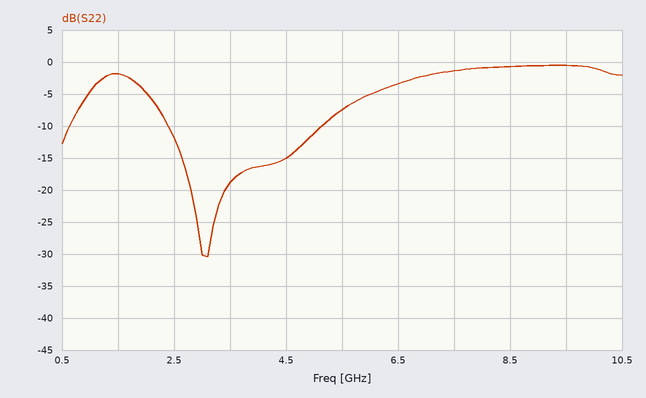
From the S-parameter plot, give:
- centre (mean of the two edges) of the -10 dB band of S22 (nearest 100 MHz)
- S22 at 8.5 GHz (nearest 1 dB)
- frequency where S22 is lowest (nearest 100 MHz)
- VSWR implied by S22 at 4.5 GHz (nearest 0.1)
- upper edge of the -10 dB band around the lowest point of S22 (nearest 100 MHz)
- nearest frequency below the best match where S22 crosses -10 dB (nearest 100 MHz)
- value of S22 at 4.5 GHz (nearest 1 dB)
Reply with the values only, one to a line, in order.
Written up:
3.8 GHz
-1 dB
3.1 GHz
1.4
5.1 GHz
2.4 GHz
-15 dB
